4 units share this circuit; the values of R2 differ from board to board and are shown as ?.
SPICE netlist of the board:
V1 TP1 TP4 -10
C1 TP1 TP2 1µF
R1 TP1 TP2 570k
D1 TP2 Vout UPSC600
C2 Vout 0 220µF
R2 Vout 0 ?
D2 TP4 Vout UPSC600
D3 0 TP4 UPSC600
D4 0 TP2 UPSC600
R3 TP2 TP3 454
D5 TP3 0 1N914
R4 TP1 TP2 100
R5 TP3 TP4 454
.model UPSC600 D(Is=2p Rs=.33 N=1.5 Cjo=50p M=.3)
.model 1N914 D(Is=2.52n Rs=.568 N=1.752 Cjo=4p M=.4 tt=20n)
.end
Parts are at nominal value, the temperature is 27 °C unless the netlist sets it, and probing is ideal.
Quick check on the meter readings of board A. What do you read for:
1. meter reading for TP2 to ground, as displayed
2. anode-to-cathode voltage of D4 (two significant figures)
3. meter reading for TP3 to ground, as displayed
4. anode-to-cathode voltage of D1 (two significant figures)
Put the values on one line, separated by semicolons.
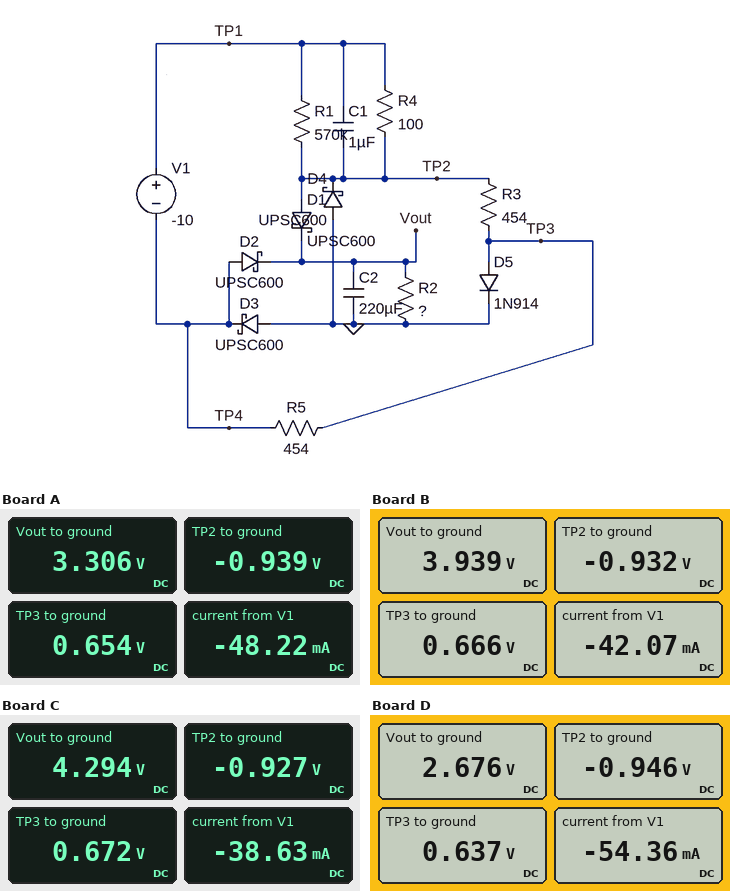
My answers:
-0.939 V; 940 mV; 0.654 V; -4.2 V
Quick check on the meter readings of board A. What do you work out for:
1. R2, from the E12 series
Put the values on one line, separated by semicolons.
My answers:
82 Ω
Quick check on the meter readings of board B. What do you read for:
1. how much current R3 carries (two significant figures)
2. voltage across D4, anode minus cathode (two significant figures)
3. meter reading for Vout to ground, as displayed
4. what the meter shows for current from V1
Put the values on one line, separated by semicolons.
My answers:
3.5 mA; 930 mV; 3.939 V; -42.07 mA
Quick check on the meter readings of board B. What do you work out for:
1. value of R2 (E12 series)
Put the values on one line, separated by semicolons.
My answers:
120 Ω
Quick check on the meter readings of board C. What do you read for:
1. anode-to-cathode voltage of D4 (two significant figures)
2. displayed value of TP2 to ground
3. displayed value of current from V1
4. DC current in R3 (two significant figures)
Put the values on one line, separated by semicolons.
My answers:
930 mV; -0.927 V; -38.63 mA; 3.5 mA
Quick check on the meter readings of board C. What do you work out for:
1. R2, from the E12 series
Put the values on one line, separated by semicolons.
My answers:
150 Ω
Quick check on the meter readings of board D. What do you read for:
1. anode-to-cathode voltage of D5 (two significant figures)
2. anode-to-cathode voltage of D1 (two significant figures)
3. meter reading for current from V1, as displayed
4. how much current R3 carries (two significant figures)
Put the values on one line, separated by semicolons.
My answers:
640 mV; -3.6 V; -54.36 mA; 3.5 mA
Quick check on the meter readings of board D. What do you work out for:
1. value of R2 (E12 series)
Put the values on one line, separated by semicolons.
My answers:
56 Ω
